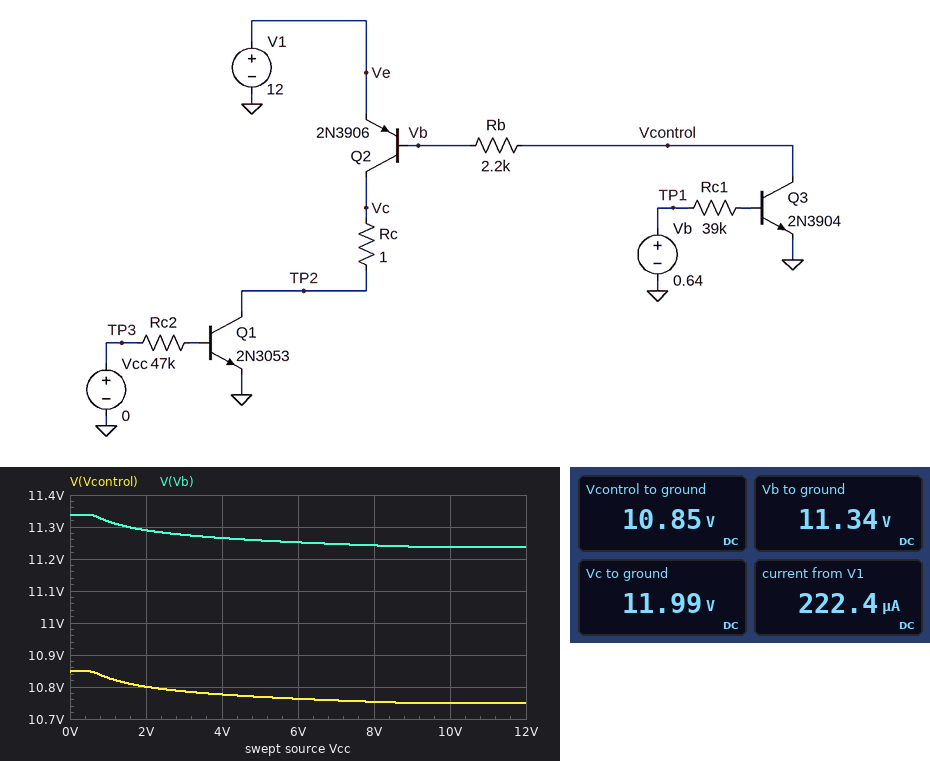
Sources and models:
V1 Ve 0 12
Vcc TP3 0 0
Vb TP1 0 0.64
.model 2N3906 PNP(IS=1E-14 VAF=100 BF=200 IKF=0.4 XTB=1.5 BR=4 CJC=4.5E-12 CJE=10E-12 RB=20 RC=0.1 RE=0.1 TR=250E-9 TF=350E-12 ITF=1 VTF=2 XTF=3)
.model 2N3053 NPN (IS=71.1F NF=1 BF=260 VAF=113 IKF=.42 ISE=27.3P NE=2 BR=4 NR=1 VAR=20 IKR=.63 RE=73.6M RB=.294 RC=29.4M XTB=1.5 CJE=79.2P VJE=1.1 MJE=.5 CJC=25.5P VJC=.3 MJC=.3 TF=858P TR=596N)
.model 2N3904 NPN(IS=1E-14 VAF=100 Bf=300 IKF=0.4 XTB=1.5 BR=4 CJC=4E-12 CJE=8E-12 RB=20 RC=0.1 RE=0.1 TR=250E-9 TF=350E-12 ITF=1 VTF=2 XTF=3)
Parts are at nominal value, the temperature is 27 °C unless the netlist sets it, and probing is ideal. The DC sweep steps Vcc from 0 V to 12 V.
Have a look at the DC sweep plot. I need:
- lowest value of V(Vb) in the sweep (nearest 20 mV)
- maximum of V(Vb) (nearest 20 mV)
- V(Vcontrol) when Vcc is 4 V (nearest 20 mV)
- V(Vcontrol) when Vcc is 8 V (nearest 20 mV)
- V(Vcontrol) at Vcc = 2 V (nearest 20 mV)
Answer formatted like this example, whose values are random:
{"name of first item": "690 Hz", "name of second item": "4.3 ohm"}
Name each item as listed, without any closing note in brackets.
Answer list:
{"lowest value of V(Vb) in the sweep": "11.24 V", "maximum of V(Vb)": "11.34 V", "V(Vcontrol) when Vcc is 4 V": "10.78 V", "V(Vcontrol) when Vcc is 8 V": "10.76 V", "V(Vcontrol) at Vcc = 2 V": "10.80 V"}
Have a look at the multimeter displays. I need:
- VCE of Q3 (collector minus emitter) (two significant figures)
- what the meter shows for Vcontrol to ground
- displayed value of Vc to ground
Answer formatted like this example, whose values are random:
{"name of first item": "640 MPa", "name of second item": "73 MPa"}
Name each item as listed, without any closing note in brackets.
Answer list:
{"VCE of Q3 (collector minus emitter)": "11 V", "what the meter shows for Vcontrol to ground": "10.85 V", "displayed value of Vc to ground": "11.99 V"}
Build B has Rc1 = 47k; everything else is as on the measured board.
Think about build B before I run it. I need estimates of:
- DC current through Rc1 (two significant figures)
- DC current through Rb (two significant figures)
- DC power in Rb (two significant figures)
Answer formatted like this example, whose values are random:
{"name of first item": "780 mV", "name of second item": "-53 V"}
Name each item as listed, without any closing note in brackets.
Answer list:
{"DC current through Rc1": "610 nA", "DC current through Rb": "200 µA", "DC power in Rb": "90 µW"}
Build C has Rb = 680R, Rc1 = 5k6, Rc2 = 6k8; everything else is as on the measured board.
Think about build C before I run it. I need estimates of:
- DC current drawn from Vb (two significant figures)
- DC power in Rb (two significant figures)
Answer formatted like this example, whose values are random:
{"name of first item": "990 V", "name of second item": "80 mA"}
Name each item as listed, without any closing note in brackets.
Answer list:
{"DC current drawn from Vb": "1.4 µA", "DC power in Rb": "140 µW"}
